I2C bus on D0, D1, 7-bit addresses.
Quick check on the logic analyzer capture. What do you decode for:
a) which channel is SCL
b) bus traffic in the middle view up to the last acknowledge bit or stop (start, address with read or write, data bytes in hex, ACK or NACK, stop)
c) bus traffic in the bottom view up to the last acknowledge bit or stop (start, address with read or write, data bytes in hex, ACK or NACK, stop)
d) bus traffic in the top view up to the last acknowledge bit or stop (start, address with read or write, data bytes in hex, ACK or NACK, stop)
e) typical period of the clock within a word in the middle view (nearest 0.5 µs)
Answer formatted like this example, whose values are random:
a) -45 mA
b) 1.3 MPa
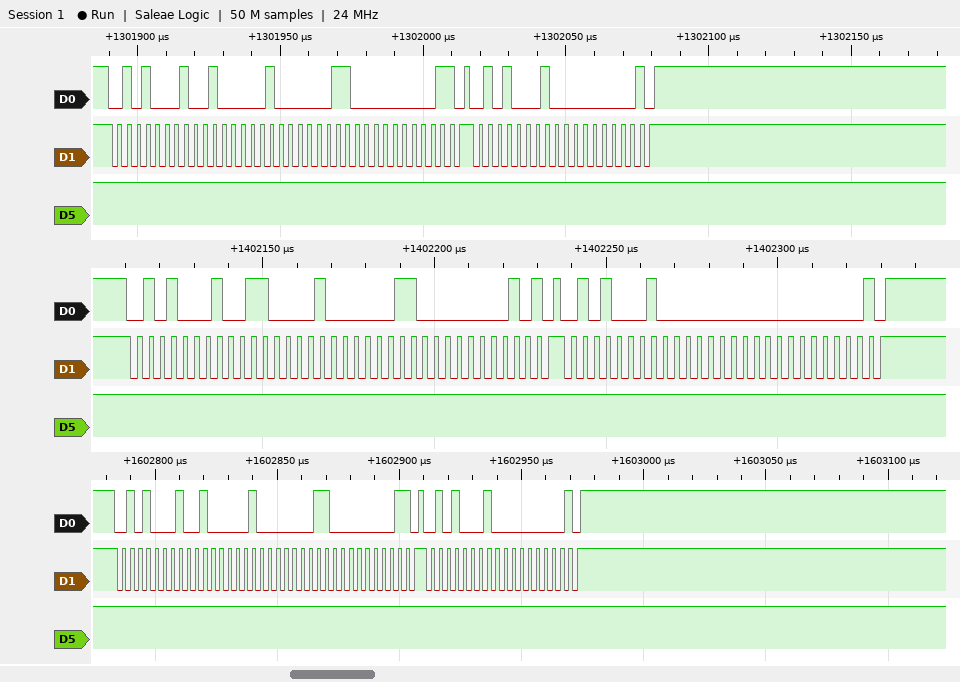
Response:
a) D1
b) start, address 28 read ACK, 61 ACK, 06 ACK, 02 NACK, stop, start, address 28 read ACK, 00 ACK, 00 NACK, stop
c) start, address 28 read ACK, 41 ACK, 03 ACK, 01 NACK, stop, start, address 28 read ACK, 00 NACK, stop
d) start, address 28 read ACK, 41 ACK, 06 ACK, 01 NACK, stop, start, address 28 read ACK, 00 NACK, stop
e) 3.5 µs
